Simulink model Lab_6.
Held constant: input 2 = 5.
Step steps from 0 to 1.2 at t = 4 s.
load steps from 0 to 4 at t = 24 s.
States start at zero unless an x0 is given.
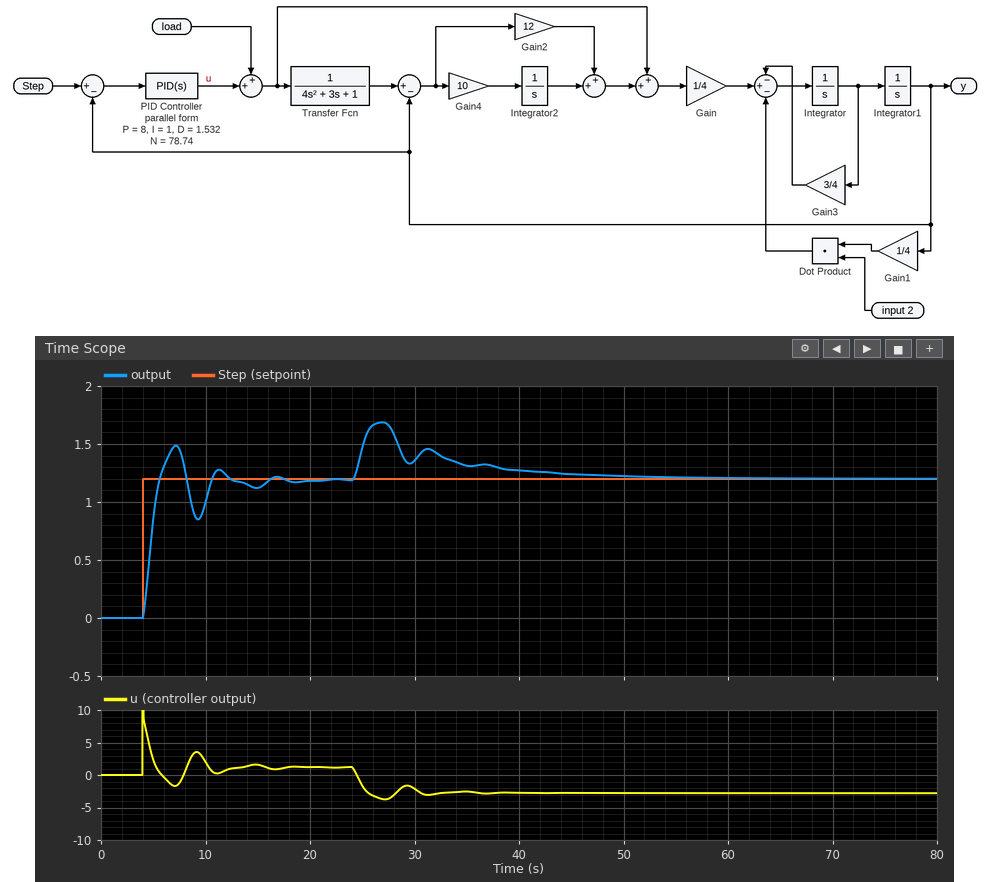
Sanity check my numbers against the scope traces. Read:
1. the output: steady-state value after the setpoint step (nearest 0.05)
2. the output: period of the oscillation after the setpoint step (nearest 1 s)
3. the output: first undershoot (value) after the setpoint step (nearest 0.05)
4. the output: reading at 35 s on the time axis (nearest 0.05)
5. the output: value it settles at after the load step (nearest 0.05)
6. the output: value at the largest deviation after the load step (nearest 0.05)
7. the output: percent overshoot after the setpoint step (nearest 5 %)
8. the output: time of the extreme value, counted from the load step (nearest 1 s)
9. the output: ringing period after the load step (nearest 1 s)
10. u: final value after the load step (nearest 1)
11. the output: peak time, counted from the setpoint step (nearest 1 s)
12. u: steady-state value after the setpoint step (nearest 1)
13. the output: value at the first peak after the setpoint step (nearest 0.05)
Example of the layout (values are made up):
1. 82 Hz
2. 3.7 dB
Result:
1. 1.20
2. 4 s
3. 0.85
4. 1.30
5. 1.20
6. 1.70
7. 25 %
8. 3 s
9. 4 s
10. -3
11. 3 s
12. 1
13. 1.50
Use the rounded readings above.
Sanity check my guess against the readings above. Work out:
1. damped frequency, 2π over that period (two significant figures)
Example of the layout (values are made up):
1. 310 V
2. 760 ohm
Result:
1. 1.6 rad/s
